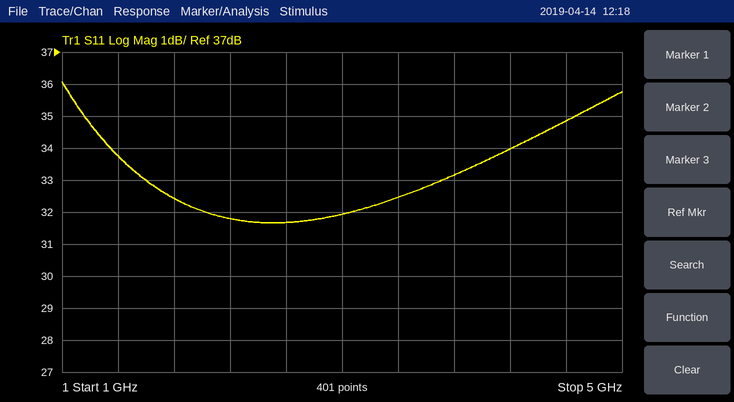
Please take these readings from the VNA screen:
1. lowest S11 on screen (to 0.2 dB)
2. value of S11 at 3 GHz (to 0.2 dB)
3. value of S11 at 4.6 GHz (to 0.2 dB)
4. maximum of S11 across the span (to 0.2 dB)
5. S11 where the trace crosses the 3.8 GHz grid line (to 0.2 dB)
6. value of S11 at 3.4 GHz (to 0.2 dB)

31.6 dB
32.0 dB
34.8 dB
36.0 dB
33.2 dB
32.4 dB
